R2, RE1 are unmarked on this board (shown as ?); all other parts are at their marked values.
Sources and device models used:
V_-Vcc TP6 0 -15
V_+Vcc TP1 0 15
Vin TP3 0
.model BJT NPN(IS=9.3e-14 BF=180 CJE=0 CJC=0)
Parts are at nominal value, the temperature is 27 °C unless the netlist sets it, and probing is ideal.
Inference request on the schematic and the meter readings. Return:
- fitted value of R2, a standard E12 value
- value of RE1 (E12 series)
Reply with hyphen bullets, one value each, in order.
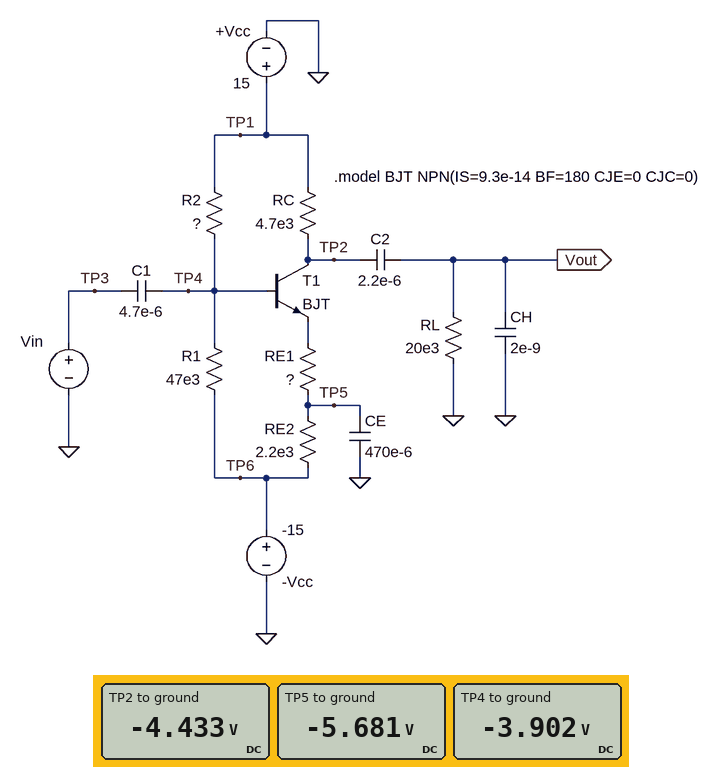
- 56 kΩ
- 270 Ω
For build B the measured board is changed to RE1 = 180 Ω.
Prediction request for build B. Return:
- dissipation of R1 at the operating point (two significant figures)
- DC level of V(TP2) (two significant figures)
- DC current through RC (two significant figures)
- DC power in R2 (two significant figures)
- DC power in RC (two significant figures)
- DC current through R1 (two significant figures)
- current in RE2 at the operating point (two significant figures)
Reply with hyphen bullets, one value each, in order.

- 2.5 mW
- -4.7 V
- 4.2 mA
- 6.5 mW
- 82 mW
- 230 µA
- 4.3 mA
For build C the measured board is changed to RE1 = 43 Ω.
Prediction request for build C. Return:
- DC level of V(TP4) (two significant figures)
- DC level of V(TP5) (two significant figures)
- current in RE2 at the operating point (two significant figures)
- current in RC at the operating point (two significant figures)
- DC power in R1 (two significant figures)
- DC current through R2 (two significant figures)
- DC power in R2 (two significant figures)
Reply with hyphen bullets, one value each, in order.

- -4.5 V
- -5.3 V
- 4.4 mA
- 4.3 mA
- 2.3 mW
- 350 µA
- 6.8 mW
